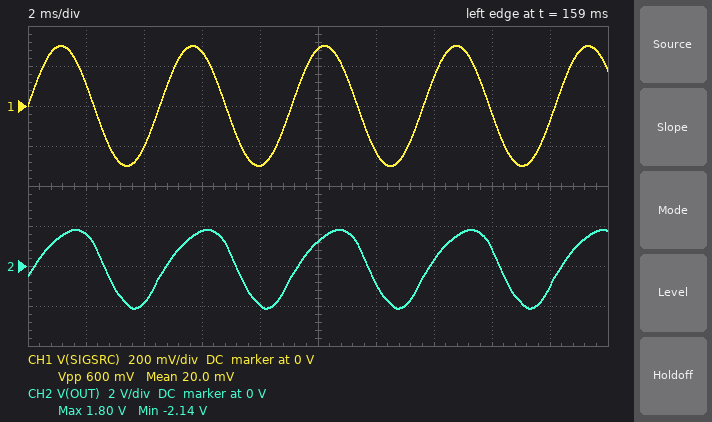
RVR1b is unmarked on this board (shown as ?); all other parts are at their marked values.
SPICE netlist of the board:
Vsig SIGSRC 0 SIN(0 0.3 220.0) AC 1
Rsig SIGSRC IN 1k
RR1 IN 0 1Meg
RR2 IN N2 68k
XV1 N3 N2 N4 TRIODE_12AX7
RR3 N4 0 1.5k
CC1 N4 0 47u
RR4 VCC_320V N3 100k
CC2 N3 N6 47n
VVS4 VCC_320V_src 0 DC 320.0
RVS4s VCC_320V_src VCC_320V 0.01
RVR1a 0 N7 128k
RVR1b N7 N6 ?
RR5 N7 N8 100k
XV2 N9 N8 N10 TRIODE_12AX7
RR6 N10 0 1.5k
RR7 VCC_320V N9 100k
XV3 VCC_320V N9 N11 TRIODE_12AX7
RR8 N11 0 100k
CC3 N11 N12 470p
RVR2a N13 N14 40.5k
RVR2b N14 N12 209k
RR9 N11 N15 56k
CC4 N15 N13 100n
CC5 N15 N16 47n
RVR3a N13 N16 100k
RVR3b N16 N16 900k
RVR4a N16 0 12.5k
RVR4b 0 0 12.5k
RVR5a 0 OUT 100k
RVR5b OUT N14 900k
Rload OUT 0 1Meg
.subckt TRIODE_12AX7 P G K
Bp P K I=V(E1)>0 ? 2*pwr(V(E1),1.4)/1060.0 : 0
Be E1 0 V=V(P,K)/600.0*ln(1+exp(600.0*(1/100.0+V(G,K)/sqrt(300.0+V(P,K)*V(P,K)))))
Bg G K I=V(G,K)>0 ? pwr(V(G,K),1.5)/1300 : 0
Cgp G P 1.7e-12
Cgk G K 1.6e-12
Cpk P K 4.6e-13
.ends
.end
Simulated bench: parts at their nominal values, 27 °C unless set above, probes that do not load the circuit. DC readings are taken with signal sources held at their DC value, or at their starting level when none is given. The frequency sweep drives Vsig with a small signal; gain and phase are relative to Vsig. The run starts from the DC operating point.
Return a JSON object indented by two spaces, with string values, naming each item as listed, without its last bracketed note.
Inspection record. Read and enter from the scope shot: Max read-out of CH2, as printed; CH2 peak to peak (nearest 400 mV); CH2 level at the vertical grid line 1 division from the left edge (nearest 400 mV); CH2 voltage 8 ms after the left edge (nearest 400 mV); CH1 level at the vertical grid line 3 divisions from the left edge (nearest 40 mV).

{
  "Max read-out of CH2, as printed": "1.80 V",
  "CH2 peak to peak": "4.0 V",
  "CH2 level at the vertical grid line 1 division from the left edge": "1.6 V",
  "CH2 voltage 8 ms after the left edge": "-2.0 V",
  "CH1 level at the vertical grid line 3 divisions from the left edge": "280 mV"
}
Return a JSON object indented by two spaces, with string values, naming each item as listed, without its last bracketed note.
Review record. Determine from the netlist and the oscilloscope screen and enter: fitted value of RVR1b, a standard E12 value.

{
  "fitted value of RVR1b, a standard E12 value": "560 kΩ"
}
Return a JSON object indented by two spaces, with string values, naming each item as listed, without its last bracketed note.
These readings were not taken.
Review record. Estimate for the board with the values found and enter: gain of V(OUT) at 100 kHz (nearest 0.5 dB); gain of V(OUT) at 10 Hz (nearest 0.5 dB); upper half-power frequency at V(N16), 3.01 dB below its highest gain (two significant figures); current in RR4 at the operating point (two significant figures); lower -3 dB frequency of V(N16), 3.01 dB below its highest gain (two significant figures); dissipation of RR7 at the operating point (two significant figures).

{
  "gain of V(OUT) at 100 kHz": "-10.5 dB",
  "gain of V(OUT) at 10 Hz": "19.5 dB",
  "upper half-power frequency at V(N16), 3.01 dB below its highest gain": "13 kHz",
  "current in RR4 at the operating point": "1.0 mA",
  "lower -3 dB frequency of V(N16), 3.01 dB below its highest gain": "82 Hz",
  "dissipation of RR7 at the operating point": "110 mW"
}
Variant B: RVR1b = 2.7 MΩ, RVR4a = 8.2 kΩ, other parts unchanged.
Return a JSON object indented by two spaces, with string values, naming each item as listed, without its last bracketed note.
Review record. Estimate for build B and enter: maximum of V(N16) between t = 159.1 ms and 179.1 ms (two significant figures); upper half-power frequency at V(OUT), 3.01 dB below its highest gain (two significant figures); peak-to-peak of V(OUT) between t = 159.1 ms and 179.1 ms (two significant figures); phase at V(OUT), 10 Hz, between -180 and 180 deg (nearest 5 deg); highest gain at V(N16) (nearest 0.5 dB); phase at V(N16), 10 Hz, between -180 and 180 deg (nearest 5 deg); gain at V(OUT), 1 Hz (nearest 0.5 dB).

{
  "maximum of V(N16) between t = 159.1 ms and 179.1 ms": "2.3 V",
  "upper half-power frequency at V(OUT), 3.01 dB below its highest gain": "110 Hz",
  "peak-to-peak of V(OUT) between t = 159.1 ms and 179.1 ms": "970 mV",
  "phase at V(OUT), 10 Hz, between -180 and 180 deg": "55 deg",
  "highest gain at V(N16)": "19.5 dB",
  "phase at V(N16), 10 Hz, between -180 and 180 deg": "65 deg",
  "gain at V(OUT), 1 Hz": "-17.0 dB"
}
